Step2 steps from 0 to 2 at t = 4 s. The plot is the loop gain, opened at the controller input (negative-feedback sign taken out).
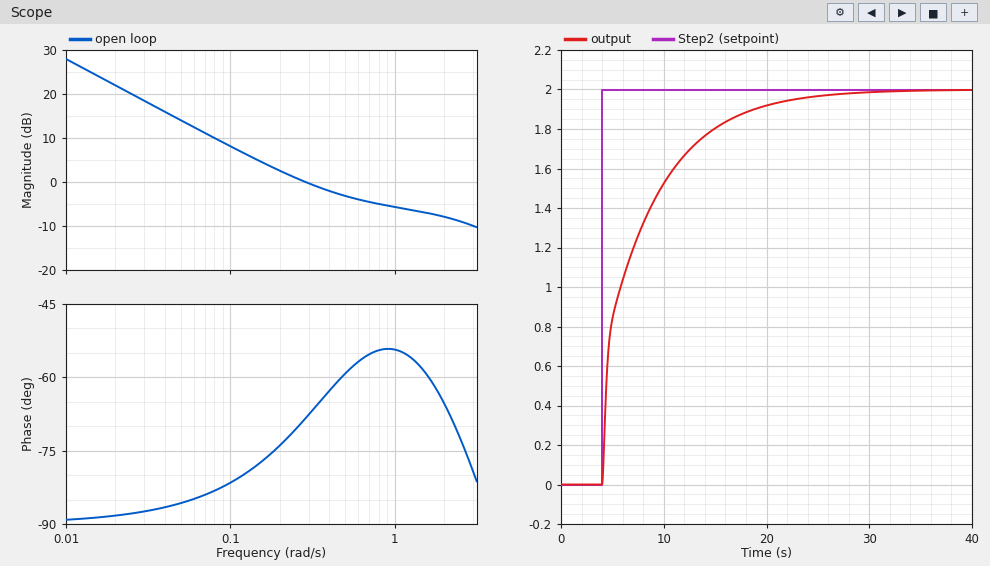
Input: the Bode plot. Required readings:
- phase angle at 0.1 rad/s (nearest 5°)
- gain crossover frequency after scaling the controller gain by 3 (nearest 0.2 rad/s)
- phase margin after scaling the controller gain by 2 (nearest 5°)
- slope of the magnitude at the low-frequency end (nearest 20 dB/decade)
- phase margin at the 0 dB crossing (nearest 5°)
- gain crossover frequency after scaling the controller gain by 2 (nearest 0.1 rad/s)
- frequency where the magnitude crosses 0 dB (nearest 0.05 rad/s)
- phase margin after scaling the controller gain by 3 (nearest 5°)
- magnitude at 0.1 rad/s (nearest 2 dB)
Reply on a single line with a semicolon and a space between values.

-80°; 2.8 rad/s; 125°; -20 dB/decade; 110°; 1.1 rad/s; 0.30 rad/s; 105°; 8 dB
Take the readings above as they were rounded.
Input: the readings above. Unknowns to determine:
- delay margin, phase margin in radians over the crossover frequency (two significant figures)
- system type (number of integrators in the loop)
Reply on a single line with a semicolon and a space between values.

6.4 s; 1
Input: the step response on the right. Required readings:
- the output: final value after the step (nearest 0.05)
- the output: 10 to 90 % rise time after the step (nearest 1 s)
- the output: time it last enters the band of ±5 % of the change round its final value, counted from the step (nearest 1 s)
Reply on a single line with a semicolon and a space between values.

2.00; 11 s; 15 s
